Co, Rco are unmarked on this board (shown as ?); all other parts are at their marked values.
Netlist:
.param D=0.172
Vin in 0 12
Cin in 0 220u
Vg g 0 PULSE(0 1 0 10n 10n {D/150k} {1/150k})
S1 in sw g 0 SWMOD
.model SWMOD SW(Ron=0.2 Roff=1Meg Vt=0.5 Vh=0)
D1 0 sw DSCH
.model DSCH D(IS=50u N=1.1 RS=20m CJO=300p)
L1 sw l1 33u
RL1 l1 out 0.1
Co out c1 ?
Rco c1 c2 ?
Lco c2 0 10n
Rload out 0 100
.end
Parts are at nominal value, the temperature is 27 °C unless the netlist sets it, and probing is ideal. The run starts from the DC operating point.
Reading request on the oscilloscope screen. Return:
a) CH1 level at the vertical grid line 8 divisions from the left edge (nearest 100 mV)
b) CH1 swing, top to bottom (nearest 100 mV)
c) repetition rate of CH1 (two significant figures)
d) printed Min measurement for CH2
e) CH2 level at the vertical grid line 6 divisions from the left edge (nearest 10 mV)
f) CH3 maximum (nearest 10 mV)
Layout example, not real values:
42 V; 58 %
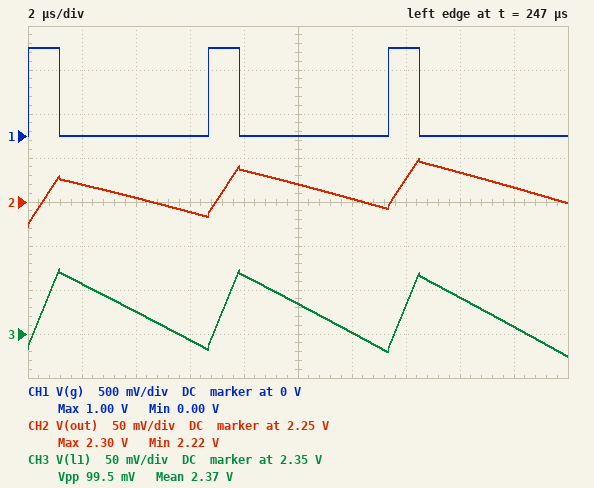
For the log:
0 V; 1.0 V; 150 kHz; 2.22 V; 2.25 V; 2.42 V
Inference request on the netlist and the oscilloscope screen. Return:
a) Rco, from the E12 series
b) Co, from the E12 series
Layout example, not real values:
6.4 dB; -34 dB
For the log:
0.15 Ω; 270 µF
